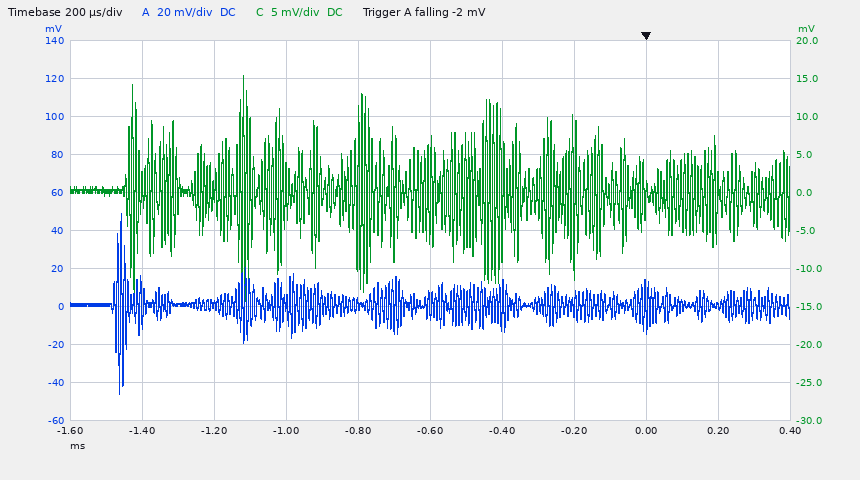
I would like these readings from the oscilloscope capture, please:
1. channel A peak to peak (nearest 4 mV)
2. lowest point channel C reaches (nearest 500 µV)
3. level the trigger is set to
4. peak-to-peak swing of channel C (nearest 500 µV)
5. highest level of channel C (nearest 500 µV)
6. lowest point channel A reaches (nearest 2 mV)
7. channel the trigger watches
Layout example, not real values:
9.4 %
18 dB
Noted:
96 mV
-14.0 mV
-2 mV
29.5 mV
15.5 mV
-46 mV
channel A
